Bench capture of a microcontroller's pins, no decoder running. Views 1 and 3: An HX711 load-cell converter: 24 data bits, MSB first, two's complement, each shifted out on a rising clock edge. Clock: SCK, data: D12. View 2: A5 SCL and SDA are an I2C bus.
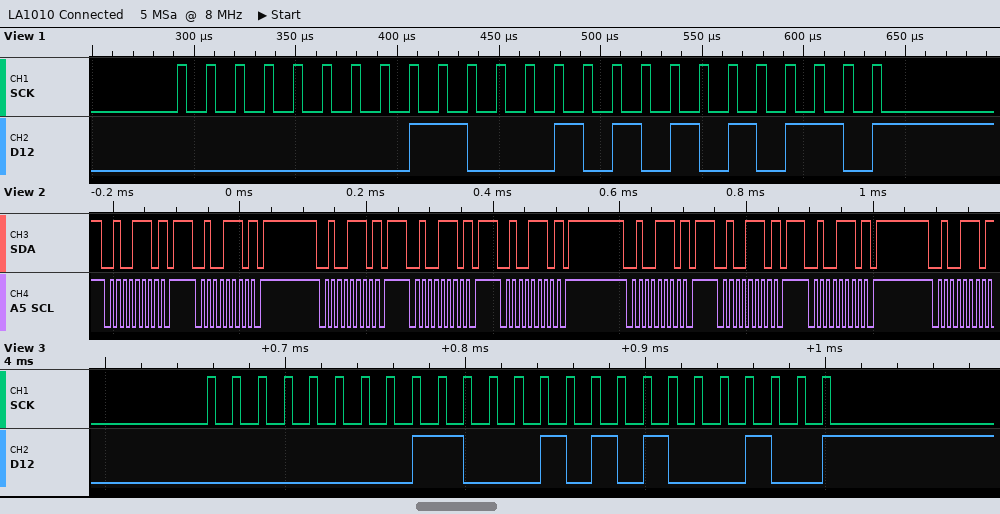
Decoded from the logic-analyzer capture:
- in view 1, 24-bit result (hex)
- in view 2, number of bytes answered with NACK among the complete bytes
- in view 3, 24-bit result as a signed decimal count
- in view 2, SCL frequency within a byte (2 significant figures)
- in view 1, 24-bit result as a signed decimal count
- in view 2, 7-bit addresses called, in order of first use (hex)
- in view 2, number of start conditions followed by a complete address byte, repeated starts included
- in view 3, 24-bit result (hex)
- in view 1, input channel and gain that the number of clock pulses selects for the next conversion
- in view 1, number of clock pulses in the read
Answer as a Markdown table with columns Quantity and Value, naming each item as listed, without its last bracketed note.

| Quantity | Value |
|---|---|
| in view 1, 24-bit result | 0x00C556 |
| in view 2, number of bytes answered with NACK among the complete bytes | 9 |
| in view 3, 24-bit result as a signed decimal count | 50500 |
| in view 2, SCL frequency within a byte | 100 kHz |
| in view 1, 24-bit result as a signed decimal count | 50518 |
| in view 2, 7-bit addresses called, in order of first use | 0x27 |
| in view 2, number of start conditions followed by a complete address byte, repeated starts included | 9 |
| in view 3, 24-bit result | 0x00C544 |
| in view 1, input channel and gain that the number of clock pulses selects for the next conversion | channel A, gain 128 |
| in view 1, number of clock pulses in the read | 25 |
